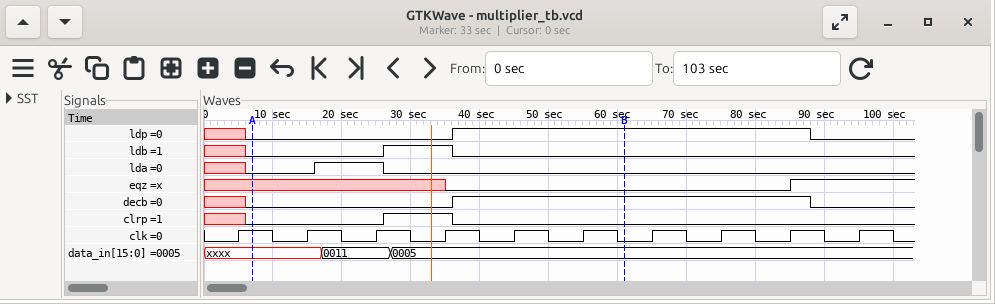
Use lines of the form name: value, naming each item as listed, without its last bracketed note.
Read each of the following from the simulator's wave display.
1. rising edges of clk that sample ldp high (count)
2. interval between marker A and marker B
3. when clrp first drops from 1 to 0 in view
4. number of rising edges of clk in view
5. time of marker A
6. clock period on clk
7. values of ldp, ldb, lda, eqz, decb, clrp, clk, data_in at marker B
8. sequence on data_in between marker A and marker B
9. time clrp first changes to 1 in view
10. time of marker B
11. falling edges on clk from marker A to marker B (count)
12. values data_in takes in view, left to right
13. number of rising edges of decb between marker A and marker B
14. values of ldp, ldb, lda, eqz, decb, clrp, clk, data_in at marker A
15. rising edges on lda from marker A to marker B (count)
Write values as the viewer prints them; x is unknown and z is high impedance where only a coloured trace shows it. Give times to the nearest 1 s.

rising edges of clk that sample ldp high: 5
interval between marker A and marker B: 54 s
when clrp first drops from 1 to 0 in view: 36 s
number of rising edges of clk in view: 10
time of marker A: 7 s
clock period on clk: 10 s
values of ldp, ldb, lda, eqz, decb, clrp, clk, data_in at marker B: ldp=1, ldb=0, lda=0, eqz=0, decb=1, clrp=0, clk=0, data_in=0005
sequence on data_in between marker A and marker B: xxxx, 0011, 0005
time clrp first changes to 1 in view: 26 s
time of marker B: 61 s
falling edges on clk from marker A to marker B: 6
values data_in takes in view, left to right: xxxx, 0011, 0005
number of rising edges of decb between marker A and marker B: 1
values of ldp, ldb, lda, eqz, decb, clrp, clk, data_in at marker A: ldp=0, ldb=0, lda=0, eqz=x, decb=0, clrp=0, clk=1, data_in=xxxx
rising edges on lda from marker A to marker B: 1
